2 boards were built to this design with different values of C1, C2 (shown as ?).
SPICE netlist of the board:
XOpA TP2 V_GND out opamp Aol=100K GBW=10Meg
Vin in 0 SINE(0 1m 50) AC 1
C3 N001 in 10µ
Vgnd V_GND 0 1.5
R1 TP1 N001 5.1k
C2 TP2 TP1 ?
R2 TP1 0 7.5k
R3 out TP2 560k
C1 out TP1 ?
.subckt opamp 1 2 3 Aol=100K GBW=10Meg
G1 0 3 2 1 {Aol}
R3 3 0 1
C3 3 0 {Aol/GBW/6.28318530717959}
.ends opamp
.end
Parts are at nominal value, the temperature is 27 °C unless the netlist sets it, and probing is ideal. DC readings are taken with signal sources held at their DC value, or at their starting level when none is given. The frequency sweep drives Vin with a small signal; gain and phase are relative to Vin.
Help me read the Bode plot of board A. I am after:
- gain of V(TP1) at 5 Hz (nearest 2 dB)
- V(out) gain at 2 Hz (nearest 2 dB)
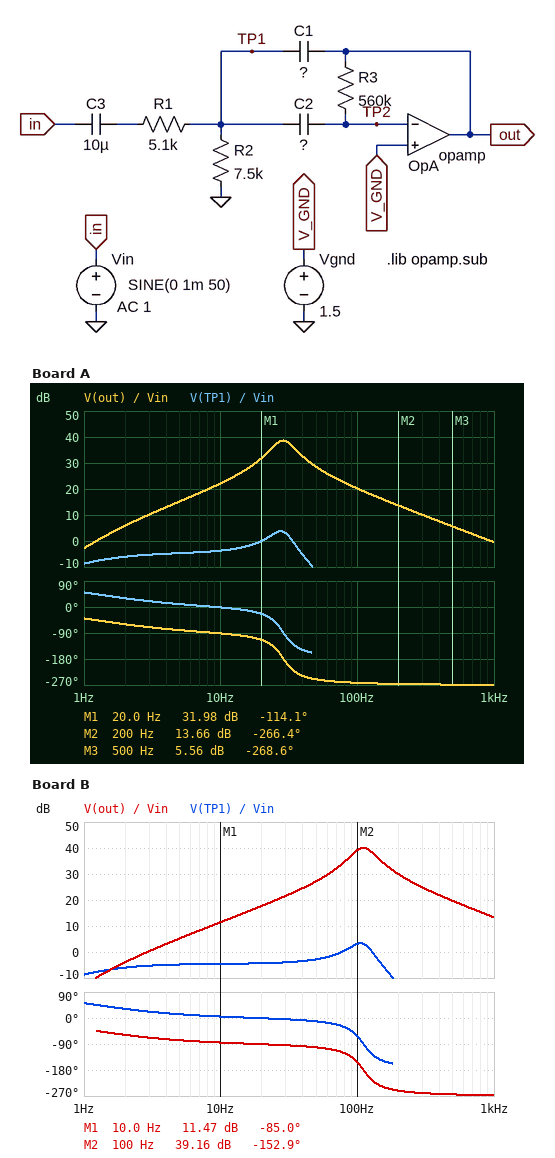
-4 dB
6 dB
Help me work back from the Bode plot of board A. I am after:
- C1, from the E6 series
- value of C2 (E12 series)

33 nF
560 nF
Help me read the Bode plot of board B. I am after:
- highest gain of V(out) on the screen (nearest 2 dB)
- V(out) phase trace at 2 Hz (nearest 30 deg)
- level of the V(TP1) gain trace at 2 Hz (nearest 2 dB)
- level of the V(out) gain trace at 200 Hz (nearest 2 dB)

40 dB
-60 deg
-6 dB
30 dB
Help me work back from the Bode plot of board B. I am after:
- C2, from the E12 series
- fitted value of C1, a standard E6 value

180 nF
6.8 nF
